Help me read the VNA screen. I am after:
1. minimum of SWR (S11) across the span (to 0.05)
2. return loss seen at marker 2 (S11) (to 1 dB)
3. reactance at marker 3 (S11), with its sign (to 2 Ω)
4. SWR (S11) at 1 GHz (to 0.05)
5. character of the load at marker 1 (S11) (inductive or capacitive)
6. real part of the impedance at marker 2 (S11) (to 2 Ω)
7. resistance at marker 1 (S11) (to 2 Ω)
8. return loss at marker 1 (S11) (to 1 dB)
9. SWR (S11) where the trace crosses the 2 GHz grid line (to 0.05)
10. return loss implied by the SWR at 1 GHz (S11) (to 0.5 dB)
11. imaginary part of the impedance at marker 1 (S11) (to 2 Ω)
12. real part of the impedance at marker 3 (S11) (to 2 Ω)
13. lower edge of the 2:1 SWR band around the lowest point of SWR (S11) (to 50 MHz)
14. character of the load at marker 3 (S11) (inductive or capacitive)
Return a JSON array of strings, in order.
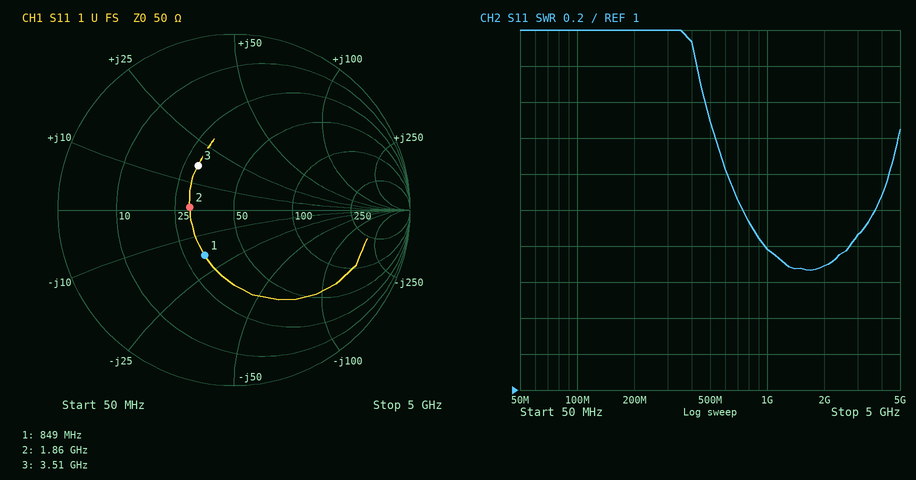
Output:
["1.65", "12 dB", "+16 Ω", "1.80", "capacitive", "30 Ω", "32 Ω", "10 dB", "1.70", "11.0 dB", "-18 Ω", "30 Ω", "750 MHz", "inductive"]
